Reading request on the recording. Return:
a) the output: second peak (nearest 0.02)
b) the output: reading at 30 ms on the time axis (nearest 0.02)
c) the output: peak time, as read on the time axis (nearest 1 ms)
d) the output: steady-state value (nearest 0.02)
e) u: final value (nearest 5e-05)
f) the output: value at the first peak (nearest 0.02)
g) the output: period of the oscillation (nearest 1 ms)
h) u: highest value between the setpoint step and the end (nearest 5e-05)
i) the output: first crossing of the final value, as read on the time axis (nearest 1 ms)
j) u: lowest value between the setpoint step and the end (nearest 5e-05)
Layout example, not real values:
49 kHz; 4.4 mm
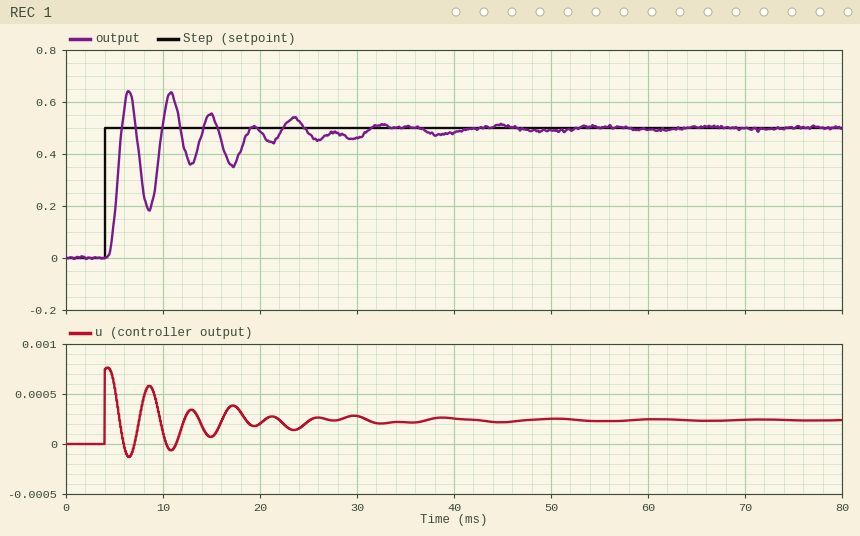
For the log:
0.64; 0.46; 6 ms; 0.50; 0.00025; 0.64; 4 ms; 0.00075; 6 ms; -0.00015
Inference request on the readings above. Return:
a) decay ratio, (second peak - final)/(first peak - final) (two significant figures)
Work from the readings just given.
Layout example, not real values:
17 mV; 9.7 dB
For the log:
1.0
